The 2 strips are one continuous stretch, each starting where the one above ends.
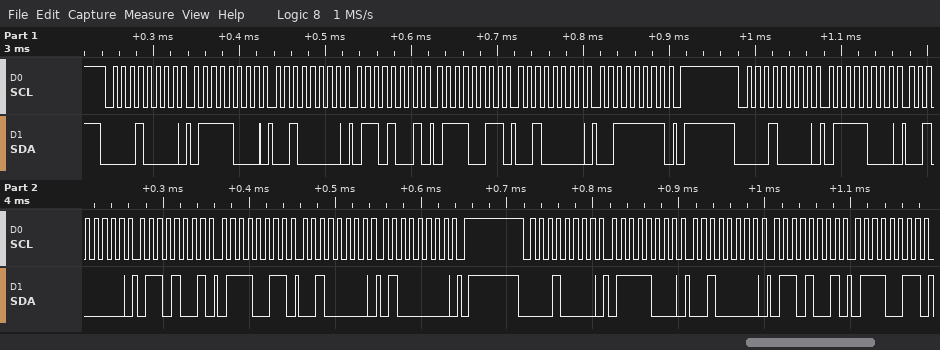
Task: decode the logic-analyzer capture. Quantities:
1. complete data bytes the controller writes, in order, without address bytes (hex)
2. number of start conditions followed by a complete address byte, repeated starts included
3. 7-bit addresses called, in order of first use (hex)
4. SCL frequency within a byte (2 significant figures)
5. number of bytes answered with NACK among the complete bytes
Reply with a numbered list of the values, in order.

1. 78 20 69 73 20 3F 78 20 69 73 20 40 78 20 69 73
2. 3
3. 0x08
4. 100 kHz
5. 0
